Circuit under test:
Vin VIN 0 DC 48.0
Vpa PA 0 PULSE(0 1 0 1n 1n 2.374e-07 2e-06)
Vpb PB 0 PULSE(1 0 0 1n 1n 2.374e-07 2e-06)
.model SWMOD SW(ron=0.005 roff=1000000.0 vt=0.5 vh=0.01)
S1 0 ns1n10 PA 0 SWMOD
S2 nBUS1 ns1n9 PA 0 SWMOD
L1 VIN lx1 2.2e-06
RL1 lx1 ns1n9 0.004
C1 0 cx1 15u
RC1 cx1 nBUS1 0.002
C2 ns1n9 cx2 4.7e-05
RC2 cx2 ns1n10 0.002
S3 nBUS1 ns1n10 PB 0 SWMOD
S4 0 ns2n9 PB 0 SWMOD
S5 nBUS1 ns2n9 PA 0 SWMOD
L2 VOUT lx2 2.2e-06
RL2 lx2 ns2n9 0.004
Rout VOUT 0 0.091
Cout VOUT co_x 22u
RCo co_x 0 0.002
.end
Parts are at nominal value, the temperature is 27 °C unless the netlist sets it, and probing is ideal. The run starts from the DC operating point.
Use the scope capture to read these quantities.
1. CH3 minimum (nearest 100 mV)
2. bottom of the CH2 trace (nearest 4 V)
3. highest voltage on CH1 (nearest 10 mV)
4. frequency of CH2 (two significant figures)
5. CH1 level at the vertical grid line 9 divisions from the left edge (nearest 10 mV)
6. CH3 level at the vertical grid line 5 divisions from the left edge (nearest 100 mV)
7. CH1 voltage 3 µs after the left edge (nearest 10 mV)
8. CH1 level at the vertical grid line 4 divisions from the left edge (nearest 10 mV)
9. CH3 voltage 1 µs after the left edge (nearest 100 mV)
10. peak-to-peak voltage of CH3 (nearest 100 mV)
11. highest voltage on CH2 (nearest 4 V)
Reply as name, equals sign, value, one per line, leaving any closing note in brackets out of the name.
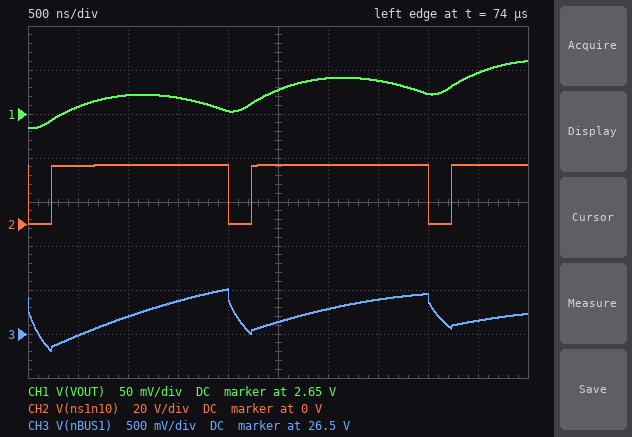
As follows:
CH3 minimum = 26.3 V
bottom of the CH2 trace = 0 V
highest voltage on CH1 = 2.71 V
frequency of CH2 = 500 kHz
CH1 level at the vertical grid line 9 divisions from the left edge = 2.70 V
CH3 level at the vertical grid line 5 divisions from the left edge = 26.6 V
CH1 voltage 3 µs after the left edge = 2.69 V
CH1 level at the vertical grid line 4 divisions from the left edge = 2.65 V
CH3 voltage 1 µs after the left edge = 26.7 V
peak-to-peak voltage of CH3 = 700 mV
highest voltage on CH2 = 28 V
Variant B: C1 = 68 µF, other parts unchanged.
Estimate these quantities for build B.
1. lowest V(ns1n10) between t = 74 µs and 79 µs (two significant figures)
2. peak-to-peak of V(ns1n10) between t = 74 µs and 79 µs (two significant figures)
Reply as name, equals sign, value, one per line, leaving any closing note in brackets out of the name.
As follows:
lowest V(ns1n10) between t = 74 µs and 79 µs = -170 mV
peak-to-peak of V(ns1n10) between t = 74 µs and 79 µs = 28 V
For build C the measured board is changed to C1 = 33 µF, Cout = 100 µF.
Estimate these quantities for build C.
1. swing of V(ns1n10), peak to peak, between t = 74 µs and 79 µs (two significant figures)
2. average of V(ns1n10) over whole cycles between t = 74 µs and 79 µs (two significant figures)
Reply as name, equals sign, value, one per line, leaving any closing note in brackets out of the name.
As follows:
swing of V(ns1n10), peak to peak, between t = 74 µs and 79 µs = 25 V
average of V(ns1n10) over whole cycles between t = 74 µs and 79 µs = 22 V
